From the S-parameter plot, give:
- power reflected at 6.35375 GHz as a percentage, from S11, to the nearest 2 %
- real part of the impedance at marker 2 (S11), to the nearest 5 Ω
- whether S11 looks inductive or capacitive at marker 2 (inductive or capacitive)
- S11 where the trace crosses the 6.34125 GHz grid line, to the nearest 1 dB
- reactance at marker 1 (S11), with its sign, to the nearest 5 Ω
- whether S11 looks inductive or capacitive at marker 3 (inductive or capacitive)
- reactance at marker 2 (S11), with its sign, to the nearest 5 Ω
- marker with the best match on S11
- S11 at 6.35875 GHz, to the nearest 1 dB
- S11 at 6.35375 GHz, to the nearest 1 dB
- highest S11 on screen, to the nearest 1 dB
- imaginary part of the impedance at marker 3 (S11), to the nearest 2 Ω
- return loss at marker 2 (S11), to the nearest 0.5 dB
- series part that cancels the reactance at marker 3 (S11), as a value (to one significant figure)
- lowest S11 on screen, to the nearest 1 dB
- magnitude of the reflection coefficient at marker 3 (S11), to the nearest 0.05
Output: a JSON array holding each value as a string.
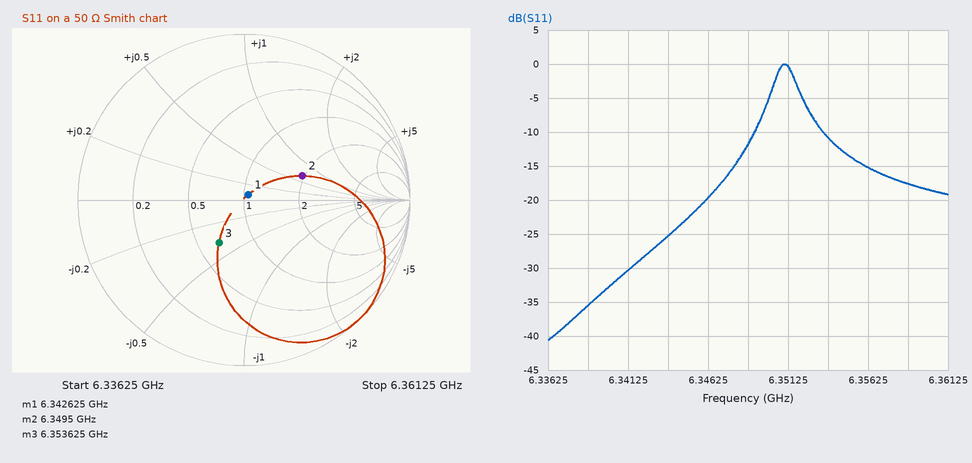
["8 %", "95 Ω", "inductive", "-30 dB", "+5 Ω", "capacitive", "+35 Ω", "marker 1", "-18 dB", "-11 dB", "0 dB", "-18 Ω", "8.5 dB", "500 pH", "-41 dB", "0.30"]
